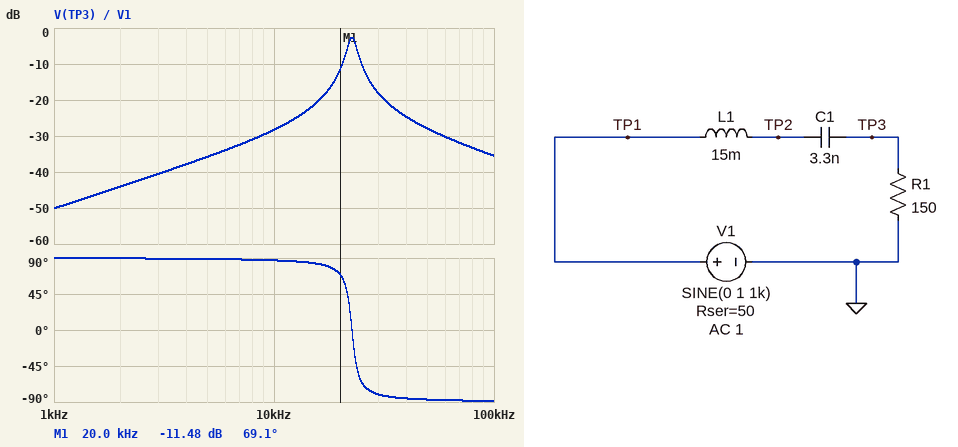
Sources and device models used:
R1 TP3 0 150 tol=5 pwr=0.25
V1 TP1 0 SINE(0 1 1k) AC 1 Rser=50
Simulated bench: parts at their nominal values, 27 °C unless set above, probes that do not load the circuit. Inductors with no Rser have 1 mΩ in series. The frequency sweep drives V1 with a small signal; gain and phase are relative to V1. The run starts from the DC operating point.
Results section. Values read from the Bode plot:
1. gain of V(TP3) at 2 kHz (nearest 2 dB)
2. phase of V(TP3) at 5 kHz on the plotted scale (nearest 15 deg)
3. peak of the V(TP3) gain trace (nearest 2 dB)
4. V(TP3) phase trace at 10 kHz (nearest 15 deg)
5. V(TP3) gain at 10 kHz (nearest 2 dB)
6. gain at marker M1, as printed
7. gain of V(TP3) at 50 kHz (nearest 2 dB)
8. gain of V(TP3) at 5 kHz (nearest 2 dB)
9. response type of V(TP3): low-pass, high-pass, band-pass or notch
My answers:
-44 dB
90 deg
-2 dB
90 deg
-28 dB
-11.48 dB
-28 dB
-36 dB
band-pass
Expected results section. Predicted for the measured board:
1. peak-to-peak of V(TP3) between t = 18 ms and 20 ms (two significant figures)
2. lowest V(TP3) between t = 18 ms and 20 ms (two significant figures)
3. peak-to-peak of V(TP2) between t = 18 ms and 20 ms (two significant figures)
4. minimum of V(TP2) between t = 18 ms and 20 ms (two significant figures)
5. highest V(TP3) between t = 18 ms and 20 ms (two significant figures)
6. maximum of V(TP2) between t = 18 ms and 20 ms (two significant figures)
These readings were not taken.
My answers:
6.2 mV
-3.1 mV
2.0 V
-1.0 V
3.1 mV
1.0 V
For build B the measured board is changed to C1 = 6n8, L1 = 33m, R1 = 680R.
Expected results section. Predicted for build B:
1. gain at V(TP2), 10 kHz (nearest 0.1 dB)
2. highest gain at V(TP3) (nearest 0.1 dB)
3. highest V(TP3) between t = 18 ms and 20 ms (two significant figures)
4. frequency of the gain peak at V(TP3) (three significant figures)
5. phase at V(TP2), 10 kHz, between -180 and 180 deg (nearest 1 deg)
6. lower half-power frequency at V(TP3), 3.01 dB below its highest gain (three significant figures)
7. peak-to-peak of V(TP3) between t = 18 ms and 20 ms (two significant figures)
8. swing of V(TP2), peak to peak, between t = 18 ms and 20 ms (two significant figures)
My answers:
9.9 dB
-0.6 dB
29 mV
10.6 kHz
-54 deg
9.01 kHz
59 mV
2.0 V
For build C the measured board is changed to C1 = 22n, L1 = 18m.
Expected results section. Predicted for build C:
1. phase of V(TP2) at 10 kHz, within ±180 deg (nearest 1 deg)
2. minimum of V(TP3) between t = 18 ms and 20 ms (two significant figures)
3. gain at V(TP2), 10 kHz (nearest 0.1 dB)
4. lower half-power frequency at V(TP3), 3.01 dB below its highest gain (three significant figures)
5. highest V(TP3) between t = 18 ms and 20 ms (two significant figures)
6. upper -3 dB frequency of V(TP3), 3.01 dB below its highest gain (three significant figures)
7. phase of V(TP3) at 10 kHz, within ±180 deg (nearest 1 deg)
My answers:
-142 deg
-21 mV
4.2 dB
7.16 kHz
21 mV
8.93 kHz
-64 deg
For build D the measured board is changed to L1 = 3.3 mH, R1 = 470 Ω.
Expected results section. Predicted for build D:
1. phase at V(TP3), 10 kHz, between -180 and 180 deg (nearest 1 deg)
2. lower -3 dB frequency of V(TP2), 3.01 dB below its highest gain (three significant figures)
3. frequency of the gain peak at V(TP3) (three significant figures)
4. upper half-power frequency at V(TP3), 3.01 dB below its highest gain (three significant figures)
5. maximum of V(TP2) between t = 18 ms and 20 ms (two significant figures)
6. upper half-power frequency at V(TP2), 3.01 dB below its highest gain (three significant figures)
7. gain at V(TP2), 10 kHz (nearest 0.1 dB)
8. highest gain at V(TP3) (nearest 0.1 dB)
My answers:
84 deg
30.8 kHz
48.2 kHz
62.4 kHz
1.0 V
57.4 kHz
0.4 dB
-0.9 dB
